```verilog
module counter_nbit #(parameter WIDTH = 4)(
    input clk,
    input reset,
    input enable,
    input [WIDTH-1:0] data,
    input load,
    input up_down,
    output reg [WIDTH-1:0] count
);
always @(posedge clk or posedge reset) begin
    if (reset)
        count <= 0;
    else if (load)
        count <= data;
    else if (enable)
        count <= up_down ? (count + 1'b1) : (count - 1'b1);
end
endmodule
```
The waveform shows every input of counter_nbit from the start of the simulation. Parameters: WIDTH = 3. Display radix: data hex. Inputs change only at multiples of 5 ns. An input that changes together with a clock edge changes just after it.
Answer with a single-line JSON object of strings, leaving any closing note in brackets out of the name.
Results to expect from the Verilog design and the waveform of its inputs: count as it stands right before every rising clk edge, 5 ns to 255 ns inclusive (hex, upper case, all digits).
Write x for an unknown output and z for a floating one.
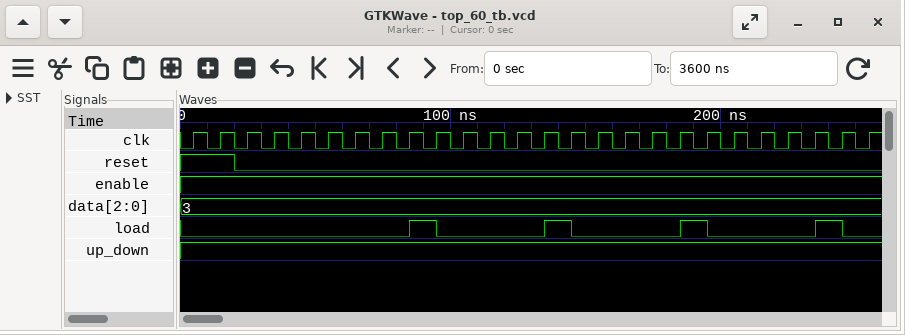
{"count as it stands right before every rising clk edge, 5 ns to 255 ns inclusive": "0, 0, 0, 1, 2, 3, 4, 5, 6, 7, 3, 4, 5, 6, 7, 3, 4, 5, 6, 7, 3, 4, 5, 6, 7, 3"}
